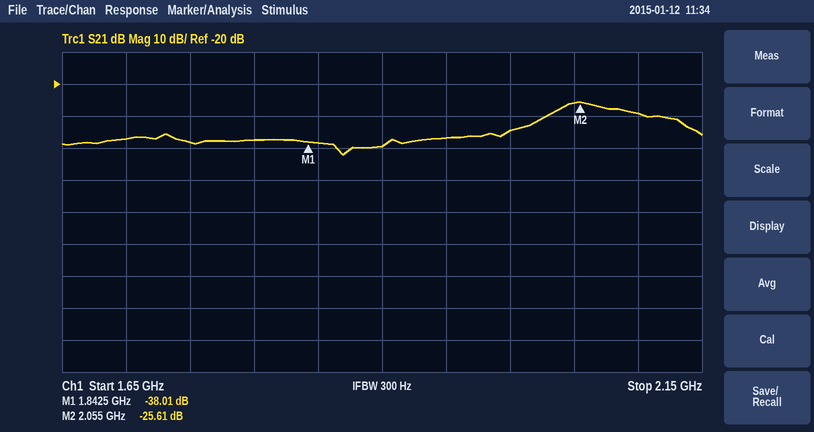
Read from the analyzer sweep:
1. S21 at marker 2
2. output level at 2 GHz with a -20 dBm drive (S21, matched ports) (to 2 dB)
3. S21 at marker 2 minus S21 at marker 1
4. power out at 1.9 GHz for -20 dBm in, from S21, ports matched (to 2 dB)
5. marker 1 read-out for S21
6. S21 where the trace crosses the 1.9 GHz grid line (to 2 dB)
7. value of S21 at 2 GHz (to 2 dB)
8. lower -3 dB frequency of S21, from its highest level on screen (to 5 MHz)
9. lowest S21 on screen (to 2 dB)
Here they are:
-25.61 dB
-54 dBm
12.40 dB
-60 dBm
-38.01 dB
-40 dB
-34 dB
2.035 GHz
-42 dB
